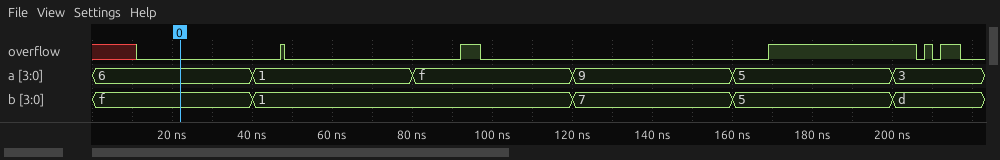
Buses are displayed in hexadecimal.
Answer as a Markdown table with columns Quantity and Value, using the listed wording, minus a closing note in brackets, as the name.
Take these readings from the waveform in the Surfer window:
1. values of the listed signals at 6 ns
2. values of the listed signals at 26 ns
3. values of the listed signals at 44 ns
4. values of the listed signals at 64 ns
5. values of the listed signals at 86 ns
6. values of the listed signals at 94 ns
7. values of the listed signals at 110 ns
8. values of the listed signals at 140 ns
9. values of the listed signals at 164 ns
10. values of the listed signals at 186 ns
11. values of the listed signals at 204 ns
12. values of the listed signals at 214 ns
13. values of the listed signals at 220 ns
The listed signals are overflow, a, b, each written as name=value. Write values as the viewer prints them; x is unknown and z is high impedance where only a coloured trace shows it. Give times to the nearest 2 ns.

| Quantity | Value |
|---|---|
| values of the listed signals at 6 ns | overflow=x, a=6, b=f |
| values of the listed signals at 26 ns | overflow=0, a=6, b=f |
| values of the listed signals at 44 ns | overflow=0, a=1, b=1 |
| values of the listed signals at 64 ns | overflow=0, a=1, b=1 |
| values of the listed signals at 86 ns | overflow=0, a=f, b=1 |
| values of the listed signals at 94 ns | overflow=1, a=f, b=1 |
| values of the listed signals at 110 ns | overflow=0, a=f, b=1 |
| values of the listed signals at 140 ns | overflow=0, a=9, b=7 |
| values of the listed signals at 164 ns | overflow=0, a=5, b=5 |
| values of the listed signals at 186 ns | overflow=1, a=5, b=5 |
| values of the listed signals at 204 ns | overflow=1, a=3, b=d |
| values of the listed signals at 214 ns | overflow=1, a=3, b=d |
| values of the listed signals at 220 ns | overflow=0, a=3, b=d |
